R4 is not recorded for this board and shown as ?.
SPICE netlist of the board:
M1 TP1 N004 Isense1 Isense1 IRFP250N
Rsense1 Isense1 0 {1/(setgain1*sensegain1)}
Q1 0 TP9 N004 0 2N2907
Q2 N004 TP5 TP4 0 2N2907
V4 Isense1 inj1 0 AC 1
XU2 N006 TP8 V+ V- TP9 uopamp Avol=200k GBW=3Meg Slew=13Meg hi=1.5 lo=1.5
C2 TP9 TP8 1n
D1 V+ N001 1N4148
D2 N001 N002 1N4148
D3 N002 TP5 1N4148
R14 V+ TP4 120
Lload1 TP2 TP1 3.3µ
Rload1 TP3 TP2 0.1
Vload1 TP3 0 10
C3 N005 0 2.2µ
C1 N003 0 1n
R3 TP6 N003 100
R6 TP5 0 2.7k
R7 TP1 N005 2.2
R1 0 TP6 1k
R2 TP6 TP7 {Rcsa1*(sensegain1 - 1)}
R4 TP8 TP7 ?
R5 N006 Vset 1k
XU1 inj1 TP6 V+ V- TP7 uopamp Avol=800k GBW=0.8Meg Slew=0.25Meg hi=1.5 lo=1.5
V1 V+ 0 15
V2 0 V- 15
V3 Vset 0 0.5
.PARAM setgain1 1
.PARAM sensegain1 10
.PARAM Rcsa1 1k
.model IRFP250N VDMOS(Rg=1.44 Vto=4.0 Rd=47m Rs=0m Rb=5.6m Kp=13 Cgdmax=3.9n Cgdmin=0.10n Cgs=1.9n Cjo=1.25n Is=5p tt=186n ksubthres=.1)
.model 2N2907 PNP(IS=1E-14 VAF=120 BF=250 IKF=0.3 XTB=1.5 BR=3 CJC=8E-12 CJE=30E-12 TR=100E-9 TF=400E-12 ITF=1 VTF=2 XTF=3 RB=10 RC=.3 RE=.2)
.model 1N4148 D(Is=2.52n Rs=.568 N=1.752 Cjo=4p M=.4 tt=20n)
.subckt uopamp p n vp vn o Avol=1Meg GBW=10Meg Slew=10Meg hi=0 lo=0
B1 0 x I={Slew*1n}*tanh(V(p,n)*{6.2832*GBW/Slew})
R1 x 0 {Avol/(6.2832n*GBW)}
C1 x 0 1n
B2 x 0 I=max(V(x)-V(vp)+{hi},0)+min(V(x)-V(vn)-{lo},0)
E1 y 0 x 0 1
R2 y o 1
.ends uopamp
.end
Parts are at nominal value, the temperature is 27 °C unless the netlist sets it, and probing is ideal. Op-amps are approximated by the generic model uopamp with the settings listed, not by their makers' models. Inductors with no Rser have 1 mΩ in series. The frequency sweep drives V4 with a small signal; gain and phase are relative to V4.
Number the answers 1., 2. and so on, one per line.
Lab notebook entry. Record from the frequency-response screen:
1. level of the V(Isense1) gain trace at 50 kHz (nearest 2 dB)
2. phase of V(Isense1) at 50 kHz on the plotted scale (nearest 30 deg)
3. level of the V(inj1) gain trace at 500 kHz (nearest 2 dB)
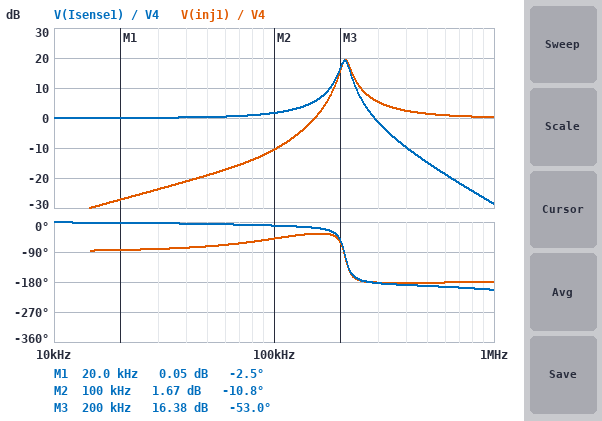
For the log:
1. 0 dB
2. 0 deg
3. 2 dB
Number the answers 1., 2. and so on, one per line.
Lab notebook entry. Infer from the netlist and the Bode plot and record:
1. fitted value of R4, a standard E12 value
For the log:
1. 820 Ω
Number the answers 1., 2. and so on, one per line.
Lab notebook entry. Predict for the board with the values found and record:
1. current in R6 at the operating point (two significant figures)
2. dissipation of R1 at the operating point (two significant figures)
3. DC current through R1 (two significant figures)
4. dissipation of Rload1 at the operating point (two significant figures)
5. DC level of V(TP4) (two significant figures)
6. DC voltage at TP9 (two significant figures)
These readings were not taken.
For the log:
1. 4.8 mA
2. 2.5 µW
3. 50 µA
4. 25 mW
5. 14 V
6. 3.6 V
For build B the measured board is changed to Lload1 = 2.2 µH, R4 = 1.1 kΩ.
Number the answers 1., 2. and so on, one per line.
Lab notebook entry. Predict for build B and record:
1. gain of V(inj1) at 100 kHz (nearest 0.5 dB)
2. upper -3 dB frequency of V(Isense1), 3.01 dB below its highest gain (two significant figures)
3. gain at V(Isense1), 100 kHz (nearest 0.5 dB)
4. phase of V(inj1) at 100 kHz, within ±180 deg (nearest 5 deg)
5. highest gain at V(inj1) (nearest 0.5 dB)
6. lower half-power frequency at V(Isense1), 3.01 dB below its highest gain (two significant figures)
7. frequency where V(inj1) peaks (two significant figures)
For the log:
1. -7.5 dB
2. 200 kHz
3. 2.0 dB
4. -55 deg
5. 15.5 dB
6. 170 kHz
7. 190 kHz
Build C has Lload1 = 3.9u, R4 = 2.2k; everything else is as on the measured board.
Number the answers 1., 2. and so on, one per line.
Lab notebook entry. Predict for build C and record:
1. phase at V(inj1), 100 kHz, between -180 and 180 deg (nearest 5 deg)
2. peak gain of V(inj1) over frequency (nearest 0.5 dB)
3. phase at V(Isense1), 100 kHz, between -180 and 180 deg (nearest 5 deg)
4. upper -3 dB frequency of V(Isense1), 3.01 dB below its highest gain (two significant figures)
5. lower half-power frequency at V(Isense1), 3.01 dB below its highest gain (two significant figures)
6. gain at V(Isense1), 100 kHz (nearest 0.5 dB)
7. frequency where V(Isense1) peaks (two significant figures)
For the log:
1. -75 deg
2. 9.0 dB
3. -40 deg
4. 160 kHz
5. 110 kHz
6. 4.0 dB
7. 140 kHz
